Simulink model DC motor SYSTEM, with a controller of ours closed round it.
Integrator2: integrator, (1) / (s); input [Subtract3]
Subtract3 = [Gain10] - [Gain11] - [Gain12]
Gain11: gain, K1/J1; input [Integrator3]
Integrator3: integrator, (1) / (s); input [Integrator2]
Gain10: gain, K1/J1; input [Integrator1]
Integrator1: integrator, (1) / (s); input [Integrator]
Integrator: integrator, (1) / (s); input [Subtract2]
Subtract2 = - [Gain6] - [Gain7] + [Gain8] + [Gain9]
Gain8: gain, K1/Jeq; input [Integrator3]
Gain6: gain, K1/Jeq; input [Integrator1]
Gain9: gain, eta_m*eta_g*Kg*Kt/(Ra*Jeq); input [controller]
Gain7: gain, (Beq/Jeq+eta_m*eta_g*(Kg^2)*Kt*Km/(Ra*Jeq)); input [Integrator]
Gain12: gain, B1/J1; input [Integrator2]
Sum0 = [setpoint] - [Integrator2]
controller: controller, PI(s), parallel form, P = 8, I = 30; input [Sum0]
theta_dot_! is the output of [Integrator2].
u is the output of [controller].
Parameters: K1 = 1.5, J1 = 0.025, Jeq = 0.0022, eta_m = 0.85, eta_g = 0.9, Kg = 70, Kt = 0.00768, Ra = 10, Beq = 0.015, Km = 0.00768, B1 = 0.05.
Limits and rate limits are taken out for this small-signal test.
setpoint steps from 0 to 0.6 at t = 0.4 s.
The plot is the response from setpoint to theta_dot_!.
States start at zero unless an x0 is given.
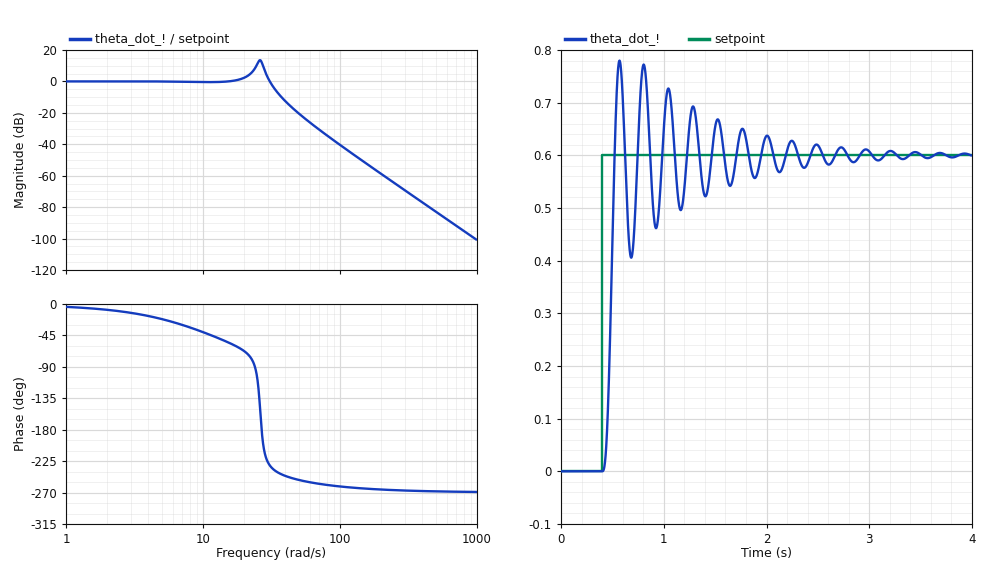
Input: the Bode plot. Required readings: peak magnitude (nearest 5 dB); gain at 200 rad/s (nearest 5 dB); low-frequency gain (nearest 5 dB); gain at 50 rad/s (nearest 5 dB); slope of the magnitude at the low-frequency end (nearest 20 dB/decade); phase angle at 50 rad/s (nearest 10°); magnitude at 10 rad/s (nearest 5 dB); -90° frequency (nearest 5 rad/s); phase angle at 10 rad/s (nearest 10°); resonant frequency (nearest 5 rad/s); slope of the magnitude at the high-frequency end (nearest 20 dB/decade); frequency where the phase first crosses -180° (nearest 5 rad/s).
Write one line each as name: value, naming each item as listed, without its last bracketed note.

peak magnitude: 15 dB
gain at 200 rad/s: -60 dB
low-frequency gain: 0 dB
gain at 50 rad/s: -20 dB
slope of the magnitude at the low-frequency end: 0 dB/decade
phase angle at 50 rad/s: -250°
magnitude at 10 rad/s: 0 dB
-90° frequency: 25 rad/s
phase angle at 10 rad/s: -40°
resonant frequency: 25 rad/s
slope of the magnitude at the high-frequency end: -60 dB/decade
frequency where the phase first crosses -180°: 25 rad/s
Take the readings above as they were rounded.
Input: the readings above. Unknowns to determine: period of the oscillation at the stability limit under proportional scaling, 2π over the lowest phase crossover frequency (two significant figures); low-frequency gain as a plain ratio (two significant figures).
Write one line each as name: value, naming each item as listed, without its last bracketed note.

period of the oscillation at the stability limit under proportional scaling, 2π over the lowest phase crossover frequency: 0.25 s
low-frequency gain as a plain ratio: 1.0
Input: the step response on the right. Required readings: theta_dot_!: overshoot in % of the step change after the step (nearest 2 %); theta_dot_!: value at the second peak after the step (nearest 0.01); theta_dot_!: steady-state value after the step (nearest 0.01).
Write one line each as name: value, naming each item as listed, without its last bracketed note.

theta_dot_!: overshoot in % of the step change after the step: 30 %
theta_dot_!: value at the second peak after the step: 0.77
theta_dot_!: steady-state value after the step: 0.60
